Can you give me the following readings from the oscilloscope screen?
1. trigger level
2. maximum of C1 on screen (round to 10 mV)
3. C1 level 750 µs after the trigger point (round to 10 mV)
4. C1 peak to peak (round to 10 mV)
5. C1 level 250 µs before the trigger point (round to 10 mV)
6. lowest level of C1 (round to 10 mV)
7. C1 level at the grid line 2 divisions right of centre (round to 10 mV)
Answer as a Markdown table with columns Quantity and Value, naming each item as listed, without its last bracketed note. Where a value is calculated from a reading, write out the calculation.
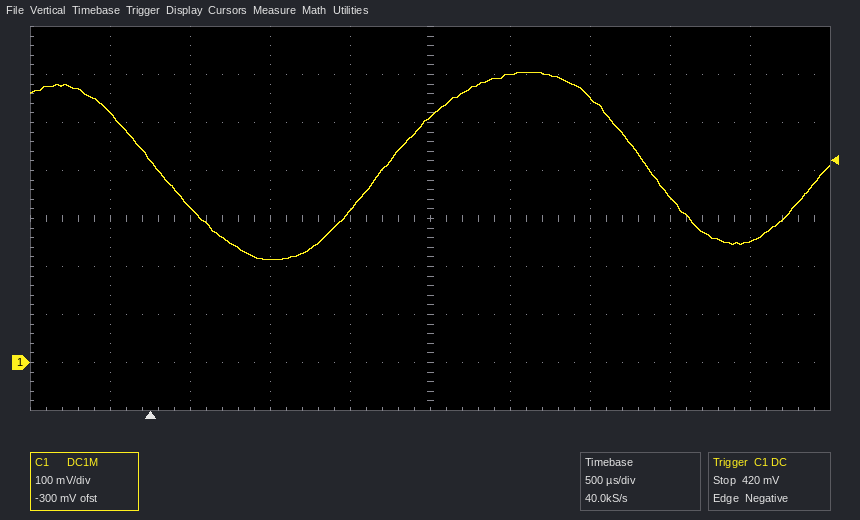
| Quantity | Value |
|---|---|
| trigger level | 420 mV |
| maximum of C1 on screen | 600 mV |
| C1 level 750 µs after the trigger point | 210 mV |
| C1 peak to peak | 600 mV − (210 mV) = 390 mV |
| C1 level 250 µs before the trigger point | 520 mV |
| lowest level of C1 | 210 mV |
| C1 level at the grid line 2 divisions right of centre | 550 mV |
